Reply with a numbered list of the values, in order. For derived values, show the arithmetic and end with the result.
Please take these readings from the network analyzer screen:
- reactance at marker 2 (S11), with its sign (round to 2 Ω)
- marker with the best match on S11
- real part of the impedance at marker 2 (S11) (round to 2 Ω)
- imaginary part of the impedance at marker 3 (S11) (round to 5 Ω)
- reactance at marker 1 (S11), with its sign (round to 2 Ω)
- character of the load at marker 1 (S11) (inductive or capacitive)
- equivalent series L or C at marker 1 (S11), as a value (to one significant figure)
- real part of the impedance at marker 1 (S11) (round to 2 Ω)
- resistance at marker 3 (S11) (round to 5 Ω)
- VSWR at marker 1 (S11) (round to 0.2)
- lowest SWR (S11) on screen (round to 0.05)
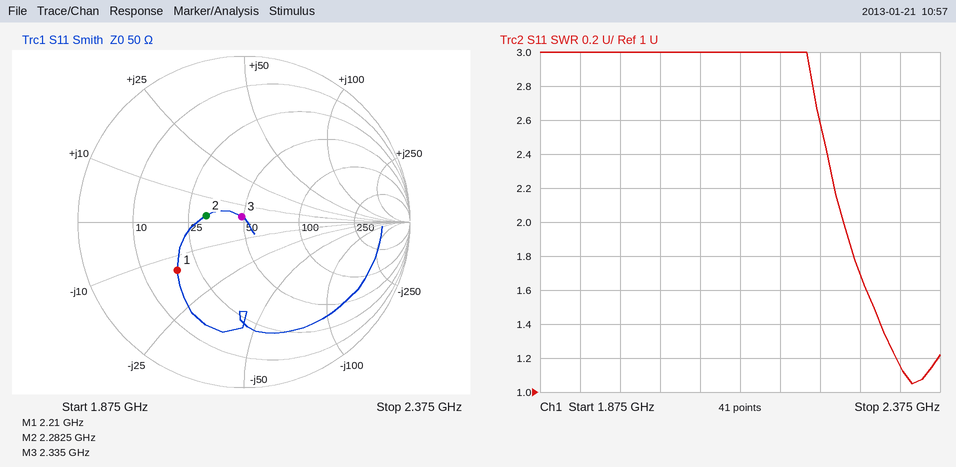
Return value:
1. +2 Ω
2. marker 3
3. 32 Ω
4. +5 Ω
5. -14 Ω
6. capacitive
7. C = 1/(2π × 2.21 GHz × 14 Ω) ≈ 5 pF
8. 18 Ω
9. 50 Ω
10. 3.0
11. 1.05
